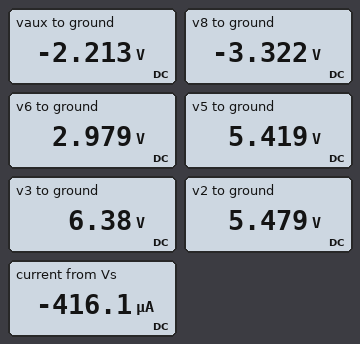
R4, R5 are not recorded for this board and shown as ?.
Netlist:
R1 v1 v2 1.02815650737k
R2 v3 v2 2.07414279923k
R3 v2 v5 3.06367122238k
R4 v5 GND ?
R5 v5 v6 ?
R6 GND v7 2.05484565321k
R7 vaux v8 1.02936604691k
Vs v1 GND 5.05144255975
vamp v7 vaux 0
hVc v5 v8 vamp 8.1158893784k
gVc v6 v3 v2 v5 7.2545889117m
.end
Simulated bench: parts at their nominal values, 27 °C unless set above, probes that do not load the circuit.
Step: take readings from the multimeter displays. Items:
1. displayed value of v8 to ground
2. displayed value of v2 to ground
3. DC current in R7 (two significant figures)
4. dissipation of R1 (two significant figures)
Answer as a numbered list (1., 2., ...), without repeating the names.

1. -3.322 V
2. 5.479 V
3. 1.1 mA
4. 180 µW
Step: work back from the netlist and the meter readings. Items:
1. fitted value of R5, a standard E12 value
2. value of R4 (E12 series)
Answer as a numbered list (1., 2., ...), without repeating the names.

1. 5.6 kΩ
2. 8.2 kΩ
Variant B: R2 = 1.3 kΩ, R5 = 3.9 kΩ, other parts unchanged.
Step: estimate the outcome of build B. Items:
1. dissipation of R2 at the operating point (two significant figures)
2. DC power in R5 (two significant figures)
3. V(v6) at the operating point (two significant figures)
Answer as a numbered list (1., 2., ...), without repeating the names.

1. 250 µW
2. 740 µW
3. 3.7 V
